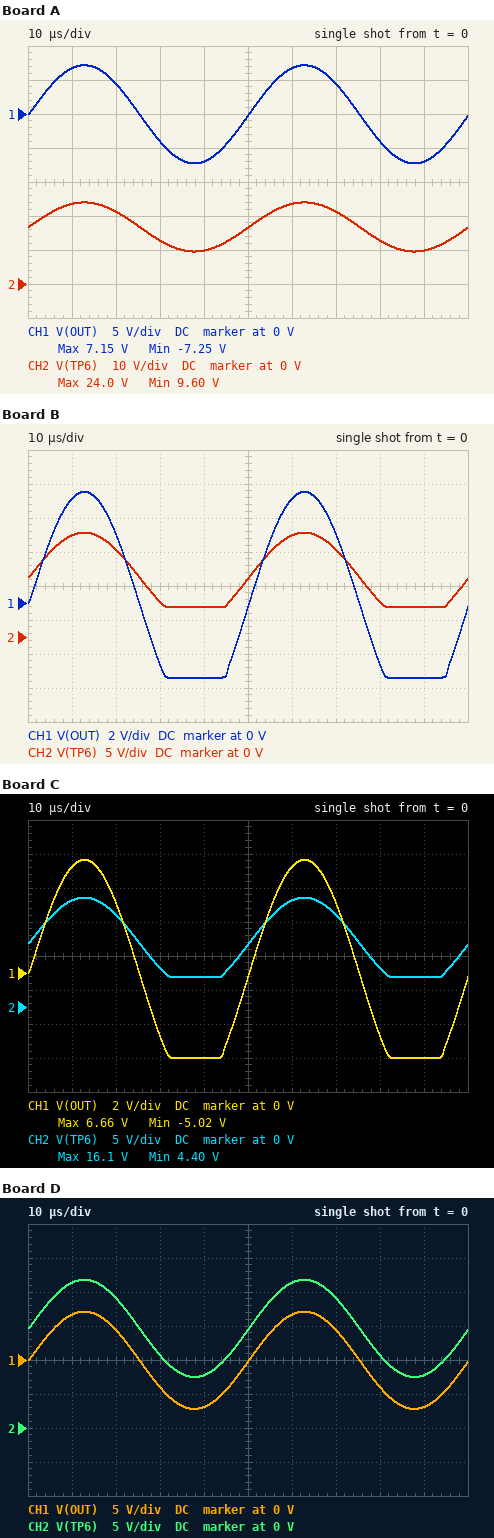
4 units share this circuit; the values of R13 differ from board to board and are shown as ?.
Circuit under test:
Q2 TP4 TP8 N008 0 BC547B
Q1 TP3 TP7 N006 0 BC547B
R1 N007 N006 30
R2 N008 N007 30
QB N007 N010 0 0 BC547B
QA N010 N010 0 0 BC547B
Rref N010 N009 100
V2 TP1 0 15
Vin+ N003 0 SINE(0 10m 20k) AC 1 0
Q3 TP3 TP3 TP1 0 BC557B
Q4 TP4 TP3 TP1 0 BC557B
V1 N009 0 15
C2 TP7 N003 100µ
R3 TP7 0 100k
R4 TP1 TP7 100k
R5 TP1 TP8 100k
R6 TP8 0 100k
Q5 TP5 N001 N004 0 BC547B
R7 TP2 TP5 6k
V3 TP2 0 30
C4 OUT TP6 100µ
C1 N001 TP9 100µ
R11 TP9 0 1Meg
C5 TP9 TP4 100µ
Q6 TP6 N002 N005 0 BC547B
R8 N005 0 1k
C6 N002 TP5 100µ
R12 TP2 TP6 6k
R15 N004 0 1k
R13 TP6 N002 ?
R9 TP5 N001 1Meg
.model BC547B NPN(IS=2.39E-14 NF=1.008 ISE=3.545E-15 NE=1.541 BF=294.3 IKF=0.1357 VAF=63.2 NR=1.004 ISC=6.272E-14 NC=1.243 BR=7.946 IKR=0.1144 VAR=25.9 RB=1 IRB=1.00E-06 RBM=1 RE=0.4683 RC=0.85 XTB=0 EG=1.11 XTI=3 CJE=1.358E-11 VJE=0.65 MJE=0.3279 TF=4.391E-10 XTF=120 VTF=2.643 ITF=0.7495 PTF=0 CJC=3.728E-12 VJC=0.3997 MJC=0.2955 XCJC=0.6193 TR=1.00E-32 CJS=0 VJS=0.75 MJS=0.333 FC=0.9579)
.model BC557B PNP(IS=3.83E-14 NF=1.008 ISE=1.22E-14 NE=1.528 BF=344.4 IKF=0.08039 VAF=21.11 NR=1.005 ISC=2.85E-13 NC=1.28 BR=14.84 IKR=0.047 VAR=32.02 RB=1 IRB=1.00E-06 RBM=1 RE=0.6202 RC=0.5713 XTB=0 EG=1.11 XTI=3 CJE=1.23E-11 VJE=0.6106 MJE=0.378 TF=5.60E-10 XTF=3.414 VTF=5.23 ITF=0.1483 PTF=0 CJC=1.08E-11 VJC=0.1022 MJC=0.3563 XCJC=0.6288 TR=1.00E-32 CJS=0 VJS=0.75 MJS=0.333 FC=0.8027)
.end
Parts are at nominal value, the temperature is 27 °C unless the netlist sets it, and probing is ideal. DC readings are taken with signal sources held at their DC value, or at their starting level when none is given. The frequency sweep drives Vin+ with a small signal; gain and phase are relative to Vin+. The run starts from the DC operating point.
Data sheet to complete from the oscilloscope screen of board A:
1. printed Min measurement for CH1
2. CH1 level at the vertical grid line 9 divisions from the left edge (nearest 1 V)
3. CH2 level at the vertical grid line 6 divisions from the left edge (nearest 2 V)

-7.25 V
-7 V
24 V
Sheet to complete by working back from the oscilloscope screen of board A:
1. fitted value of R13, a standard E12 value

2.2 MΩ
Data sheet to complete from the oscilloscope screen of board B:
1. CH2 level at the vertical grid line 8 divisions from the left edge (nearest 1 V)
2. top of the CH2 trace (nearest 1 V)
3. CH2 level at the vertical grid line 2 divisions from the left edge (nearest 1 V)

5 V
15 V
13 V
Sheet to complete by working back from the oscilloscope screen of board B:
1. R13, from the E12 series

390 kΩ
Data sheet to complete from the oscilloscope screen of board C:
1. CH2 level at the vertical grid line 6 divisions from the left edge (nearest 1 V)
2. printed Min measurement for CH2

16 V
4.40 V
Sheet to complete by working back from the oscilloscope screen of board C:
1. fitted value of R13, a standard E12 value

470 kΩ
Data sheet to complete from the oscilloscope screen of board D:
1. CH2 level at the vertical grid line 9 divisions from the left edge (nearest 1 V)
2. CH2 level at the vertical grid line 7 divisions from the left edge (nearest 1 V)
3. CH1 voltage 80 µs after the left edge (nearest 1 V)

8 V
19 V
-4 V
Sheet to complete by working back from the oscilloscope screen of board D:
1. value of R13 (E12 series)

1.5 MΩ
